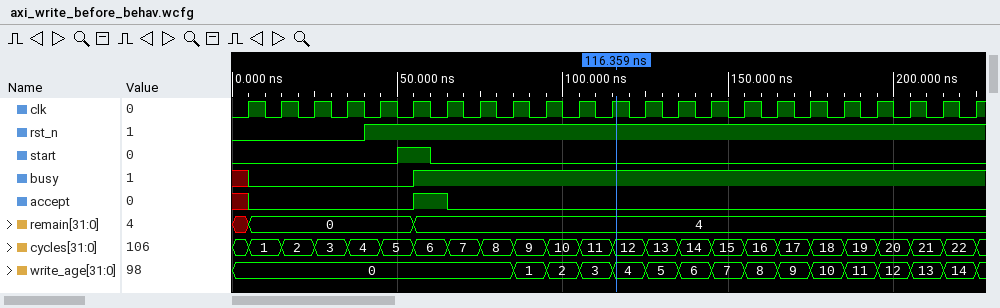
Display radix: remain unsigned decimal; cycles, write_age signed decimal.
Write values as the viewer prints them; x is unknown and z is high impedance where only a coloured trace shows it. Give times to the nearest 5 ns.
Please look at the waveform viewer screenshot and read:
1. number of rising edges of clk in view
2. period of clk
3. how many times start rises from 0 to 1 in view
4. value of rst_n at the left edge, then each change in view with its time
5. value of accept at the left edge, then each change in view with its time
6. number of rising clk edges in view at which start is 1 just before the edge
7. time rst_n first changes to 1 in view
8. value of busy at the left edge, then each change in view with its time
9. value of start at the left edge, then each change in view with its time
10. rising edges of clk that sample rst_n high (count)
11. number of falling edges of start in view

23
10 ns
1
0, 1 at 40 ns
x, 0 at 5 ns, 1 at 55 ns, 0 at 65 ns
1
40 ns
x, 0 at 5 ns, 1 at 55 ns
0, 1 at 50 ns, 0 at 60 ns
19
1
